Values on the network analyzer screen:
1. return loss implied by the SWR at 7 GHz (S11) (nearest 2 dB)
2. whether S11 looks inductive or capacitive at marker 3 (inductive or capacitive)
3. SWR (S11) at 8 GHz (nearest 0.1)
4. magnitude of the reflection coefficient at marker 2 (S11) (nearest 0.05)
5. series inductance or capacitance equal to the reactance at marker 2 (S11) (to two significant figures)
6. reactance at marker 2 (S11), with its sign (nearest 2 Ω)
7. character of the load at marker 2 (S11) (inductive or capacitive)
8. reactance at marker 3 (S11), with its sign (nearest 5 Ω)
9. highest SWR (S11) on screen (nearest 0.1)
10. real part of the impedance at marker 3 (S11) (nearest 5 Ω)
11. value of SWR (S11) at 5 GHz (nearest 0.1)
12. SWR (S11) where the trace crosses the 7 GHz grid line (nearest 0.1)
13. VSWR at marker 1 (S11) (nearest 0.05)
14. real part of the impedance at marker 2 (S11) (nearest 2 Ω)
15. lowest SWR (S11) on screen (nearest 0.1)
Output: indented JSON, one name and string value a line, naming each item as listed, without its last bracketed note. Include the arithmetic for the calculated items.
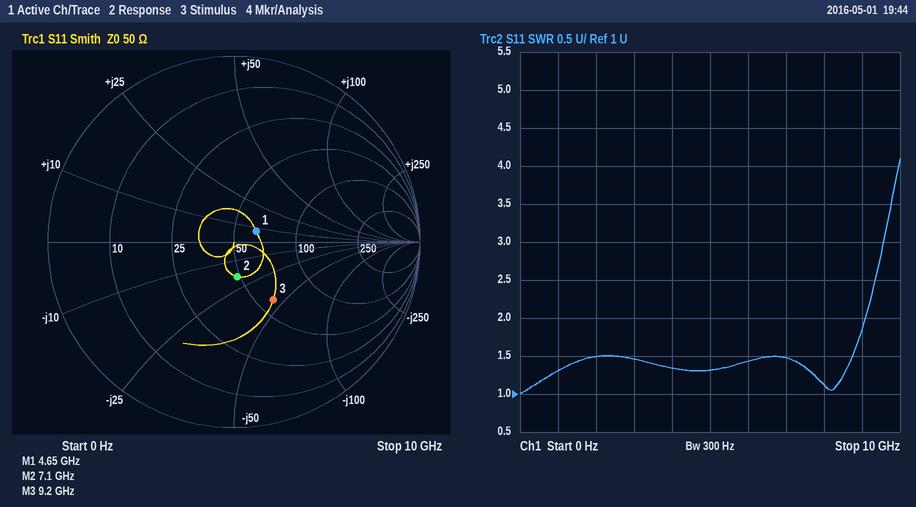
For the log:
{
  "return loss implied by the SWR at 7 GHz (S11)": "−20 log10((1.5 − 1)/(1.5 + 1)) ≈ 14 dB",
  "whether S11 looks inductive or capacitive at marker 3": "capacitive",
  "SWR (S11) at 8 GHz": "1.1",
  "magnitude of the reflection coefficient at marker 2 (S11)": "0.20",
  "series inductance or capacitance equal to the reactance at marker 2 (S11)": "C = 1/(2π × 7.1 GHz × 18 Ω) ≈ 1.2 pF",
  "reactance at marker 2 (S11), with its sign": "-18 Ω",
  "character of the load at marker 2 (S11)": "capacitive",
  "reactance at marker 3 (S11), with its sign": "-45 Ω",
  "highest SWR (S11) on screen": "4.1",
  "real part of the impedance at marker 3 (S11)": "60 Ω",
  "value of SWR (S11) at 5 GHz": "1.3",
  "SWR (S11) where the trace crosses the 7 GHz grid line": "1.5",
  "VSWR at marker 1 (S11)": "1.30",
  "real part of the impedance at marker 2 (S11)": "48 Ω",
  "lowest SWR (S11) on screen": "1.0"
}
